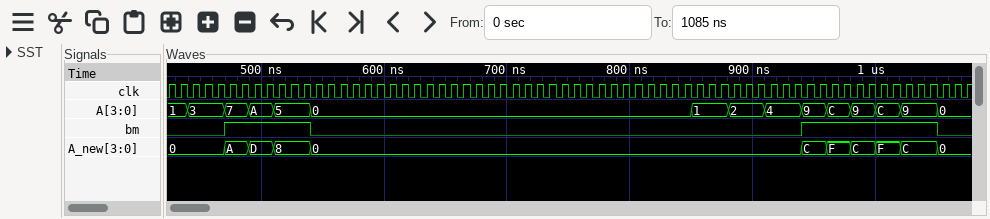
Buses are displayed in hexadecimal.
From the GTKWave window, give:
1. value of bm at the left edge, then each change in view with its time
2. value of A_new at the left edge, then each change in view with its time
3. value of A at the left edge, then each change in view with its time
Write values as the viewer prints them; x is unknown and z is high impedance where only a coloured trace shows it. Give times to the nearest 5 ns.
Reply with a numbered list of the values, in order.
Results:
1. 0, 1 at 470 ns, 0 at 540 ns, 1 at 940 ns, 0 at 1050 ns
2. 0, A at 470 ns, D at 490 ns, 8 at 510 ns, 0 at 540 ns, C at 940 ns, F at 960 ns, C at 980 ns, F at 1000 ns, C at 1020 ns, 0 at 1050 ns
3. 1, 3 at 440 ns, 7 at 470 ns, A at 490 ns, 5 at 510 ns, 0 at 540 ns, 1 at 850 ns, 2 at 880 ns, 4 at 910 ns, 9 at 940 ns, C at 960 ns, 9 at 980 ns, C at 1000 ns, 9 at 1020 ns, 0 at 1050 ns
